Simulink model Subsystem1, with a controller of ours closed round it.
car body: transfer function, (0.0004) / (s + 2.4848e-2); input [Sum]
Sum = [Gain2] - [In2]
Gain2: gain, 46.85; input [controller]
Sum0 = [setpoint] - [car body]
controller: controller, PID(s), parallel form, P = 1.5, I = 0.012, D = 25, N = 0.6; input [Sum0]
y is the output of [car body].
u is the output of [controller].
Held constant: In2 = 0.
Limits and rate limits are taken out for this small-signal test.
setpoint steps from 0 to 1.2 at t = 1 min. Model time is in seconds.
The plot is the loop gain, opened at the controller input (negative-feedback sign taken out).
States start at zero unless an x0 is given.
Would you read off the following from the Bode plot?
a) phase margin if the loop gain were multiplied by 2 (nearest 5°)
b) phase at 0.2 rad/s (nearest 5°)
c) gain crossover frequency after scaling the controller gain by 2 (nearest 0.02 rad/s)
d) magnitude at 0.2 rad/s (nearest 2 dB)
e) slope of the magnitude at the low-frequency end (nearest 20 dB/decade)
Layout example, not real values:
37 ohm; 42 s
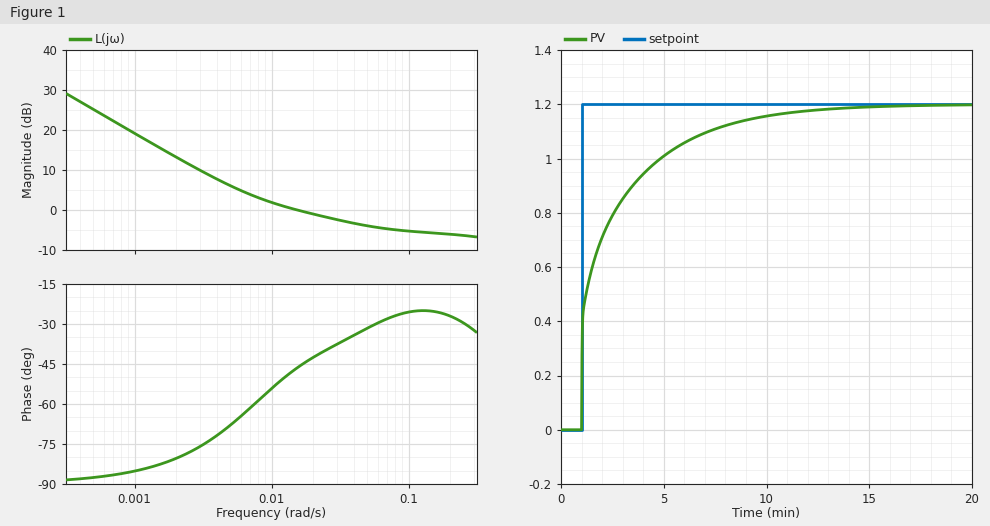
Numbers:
155°; -25°; 0.20 rad/s; -6 dB; -20 dB/decade
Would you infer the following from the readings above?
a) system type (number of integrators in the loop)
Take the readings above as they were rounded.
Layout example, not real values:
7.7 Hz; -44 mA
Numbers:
1
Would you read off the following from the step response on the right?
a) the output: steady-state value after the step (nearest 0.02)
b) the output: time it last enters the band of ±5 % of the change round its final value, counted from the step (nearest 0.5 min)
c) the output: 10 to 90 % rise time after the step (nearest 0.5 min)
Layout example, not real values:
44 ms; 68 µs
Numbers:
1.20; 8.0 min; 5.5 min
